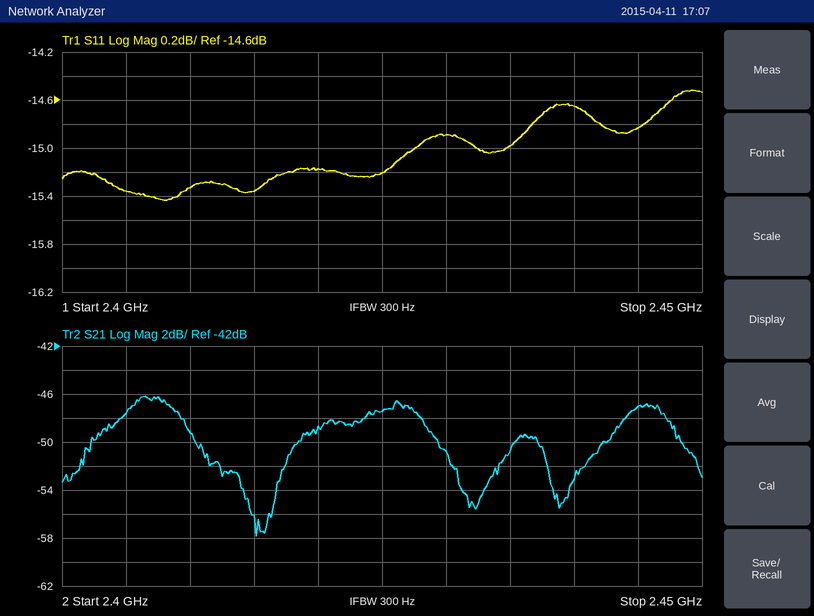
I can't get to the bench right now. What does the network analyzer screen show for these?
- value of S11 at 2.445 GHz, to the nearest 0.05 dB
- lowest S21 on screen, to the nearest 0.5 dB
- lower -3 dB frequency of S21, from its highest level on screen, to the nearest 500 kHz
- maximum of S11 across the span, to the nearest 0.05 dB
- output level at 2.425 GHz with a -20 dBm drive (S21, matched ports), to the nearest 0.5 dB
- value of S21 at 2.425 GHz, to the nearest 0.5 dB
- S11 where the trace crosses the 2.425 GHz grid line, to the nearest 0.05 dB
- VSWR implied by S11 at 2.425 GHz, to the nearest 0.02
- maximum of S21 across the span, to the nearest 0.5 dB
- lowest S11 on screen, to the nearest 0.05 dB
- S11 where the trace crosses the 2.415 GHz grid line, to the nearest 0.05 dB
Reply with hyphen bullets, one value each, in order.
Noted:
- -14.85 dB
- -58.0 dB
- 2.4030 GHz
- -14.50 dB
- -67.5 dBm
- -47.5 dB
- -15.20 dB
- 1.42
- -46.0 dB
- -15.45 dB
- -15.35 dB
